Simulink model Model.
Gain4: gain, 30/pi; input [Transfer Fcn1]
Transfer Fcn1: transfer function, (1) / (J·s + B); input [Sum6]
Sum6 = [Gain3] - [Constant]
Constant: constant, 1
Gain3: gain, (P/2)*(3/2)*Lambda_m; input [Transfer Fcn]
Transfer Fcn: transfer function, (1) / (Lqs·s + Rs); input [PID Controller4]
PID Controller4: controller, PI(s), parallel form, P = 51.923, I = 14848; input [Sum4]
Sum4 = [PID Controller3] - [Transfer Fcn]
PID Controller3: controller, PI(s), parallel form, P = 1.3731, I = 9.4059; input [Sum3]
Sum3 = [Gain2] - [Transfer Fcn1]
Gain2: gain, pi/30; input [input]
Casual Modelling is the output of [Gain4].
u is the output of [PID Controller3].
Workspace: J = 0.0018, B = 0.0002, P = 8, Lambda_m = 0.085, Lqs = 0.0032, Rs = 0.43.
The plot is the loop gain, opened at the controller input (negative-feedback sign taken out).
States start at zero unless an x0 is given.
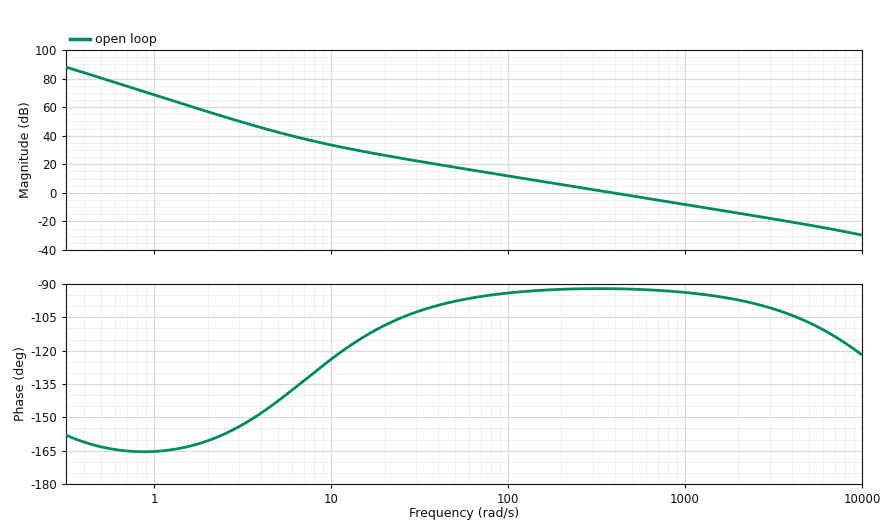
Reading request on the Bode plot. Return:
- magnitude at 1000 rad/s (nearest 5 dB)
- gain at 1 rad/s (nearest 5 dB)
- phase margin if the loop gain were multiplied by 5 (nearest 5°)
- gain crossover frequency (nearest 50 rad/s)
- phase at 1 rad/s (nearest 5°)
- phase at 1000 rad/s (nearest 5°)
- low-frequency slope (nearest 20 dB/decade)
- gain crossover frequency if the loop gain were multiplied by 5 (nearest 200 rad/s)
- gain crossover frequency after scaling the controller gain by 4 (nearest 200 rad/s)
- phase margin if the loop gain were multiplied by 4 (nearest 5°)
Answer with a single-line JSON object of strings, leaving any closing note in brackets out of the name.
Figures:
{"magnitude at 1000 rad/s": "-10 dB", "gain at 1 rad/s": "70 dB", "phase margin if the loop gain were multiplied by 5": "85°", "gain crossover frequency": "400 rad/s", "phase at 1 rad/s": "-165°", "phase at 1000 rad/s": "-95°", "low-frequency slope": "-40 dB/decade", "gain crossover frequency if the loop gain were multiplied by 5": "2000 rad/s", "gain crossover frequency after scaling the controller gain by 4": "1600 rad/s", "phase margin if the loop gain were multiplied by 4": "85°"}
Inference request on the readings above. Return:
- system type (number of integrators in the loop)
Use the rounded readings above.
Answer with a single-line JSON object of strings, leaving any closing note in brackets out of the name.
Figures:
{"system type": "2"}
